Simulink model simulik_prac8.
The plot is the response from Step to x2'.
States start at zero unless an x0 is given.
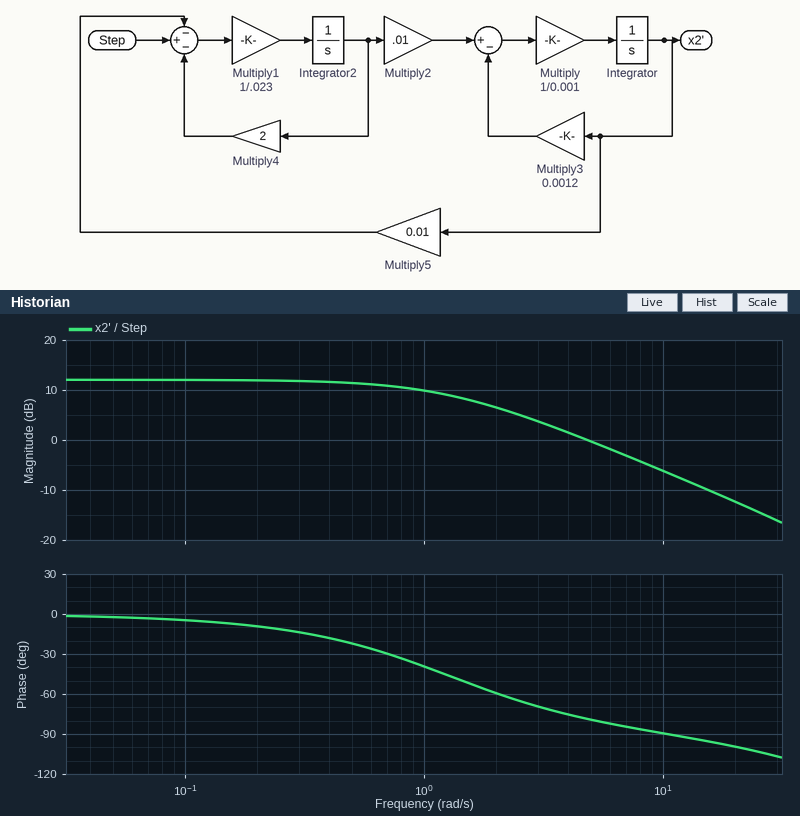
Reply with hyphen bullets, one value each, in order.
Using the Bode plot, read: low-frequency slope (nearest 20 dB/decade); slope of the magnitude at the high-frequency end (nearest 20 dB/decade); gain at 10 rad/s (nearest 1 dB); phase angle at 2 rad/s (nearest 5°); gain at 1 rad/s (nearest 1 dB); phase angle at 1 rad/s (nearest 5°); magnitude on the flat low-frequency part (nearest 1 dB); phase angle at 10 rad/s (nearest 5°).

- 0 dB/decade
- -20 dB/decade
- -6 dB
- -60°
- 10 dB
- -40°
- 12 dB
- -90°
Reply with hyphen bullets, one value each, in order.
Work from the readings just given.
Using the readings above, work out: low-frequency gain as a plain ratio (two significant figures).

- 4.0
